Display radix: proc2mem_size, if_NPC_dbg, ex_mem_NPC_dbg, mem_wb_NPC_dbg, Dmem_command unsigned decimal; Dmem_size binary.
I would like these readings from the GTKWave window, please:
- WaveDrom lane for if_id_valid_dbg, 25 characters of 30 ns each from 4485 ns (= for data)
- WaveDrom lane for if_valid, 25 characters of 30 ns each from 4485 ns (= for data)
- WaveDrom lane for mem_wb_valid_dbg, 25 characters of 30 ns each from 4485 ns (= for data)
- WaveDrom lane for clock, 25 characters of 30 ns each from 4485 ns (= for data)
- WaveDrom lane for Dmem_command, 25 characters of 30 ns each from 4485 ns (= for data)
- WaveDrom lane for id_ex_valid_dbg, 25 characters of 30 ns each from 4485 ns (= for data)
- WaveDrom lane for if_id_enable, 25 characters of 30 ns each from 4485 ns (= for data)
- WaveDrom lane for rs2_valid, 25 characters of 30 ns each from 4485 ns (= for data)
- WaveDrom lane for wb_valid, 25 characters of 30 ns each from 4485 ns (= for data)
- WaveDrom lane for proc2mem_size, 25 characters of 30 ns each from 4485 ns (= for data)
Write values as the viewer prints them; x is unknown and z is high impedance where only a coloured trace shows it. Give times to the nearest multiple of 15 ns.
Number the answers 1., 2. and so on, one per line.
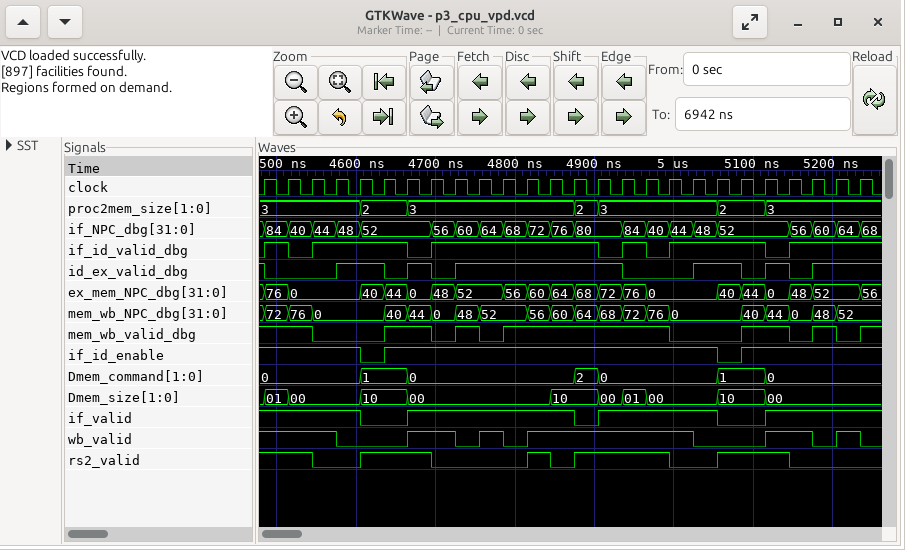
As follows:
1. {name: 'if_id_valid_dbg', wave: '101...01......0101...01..'}
2. {name: 'if_valid', wave: '1...0.1......01....0.1...'}
3. {name: 'mem_wb_valid_dbg', wave: '1.0..1.0101......0..1.010'}
4. {name: 'clock', wave: 'p........................'}
5. {name: 'Dmem_command', wave: '=...=.=......==....=.=...', data: '0 1 0 2 0 1 0'}
6. {name: 'id_ex_valid_dbg', wave: '0..1.0101......0..1.0101.'}
7. {name: 'if_id_enable', wave: '1...01.............01....'}
8. {name: 'rs2_valid', wave: '1.0.1..0...101...0.1..0..'}
9. {name: 'wb_valid', wave: '1..0..1.0101......0..1.01'}
10. {name: 'proc2mem_size', wave: '=...=.=......==....=.=...', data: '3 2 3 2 3 2 3'}
